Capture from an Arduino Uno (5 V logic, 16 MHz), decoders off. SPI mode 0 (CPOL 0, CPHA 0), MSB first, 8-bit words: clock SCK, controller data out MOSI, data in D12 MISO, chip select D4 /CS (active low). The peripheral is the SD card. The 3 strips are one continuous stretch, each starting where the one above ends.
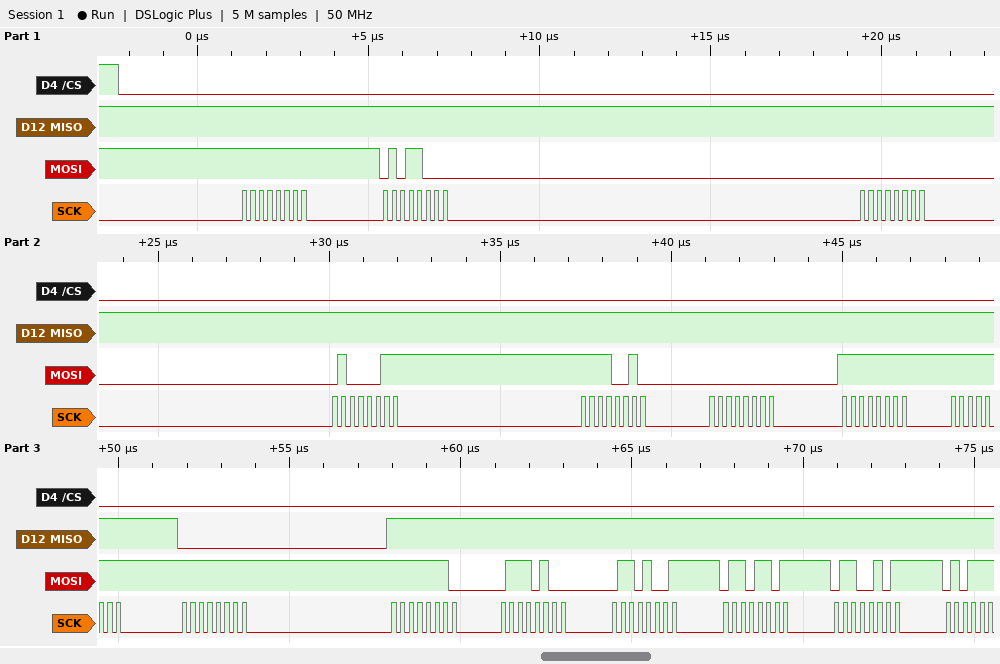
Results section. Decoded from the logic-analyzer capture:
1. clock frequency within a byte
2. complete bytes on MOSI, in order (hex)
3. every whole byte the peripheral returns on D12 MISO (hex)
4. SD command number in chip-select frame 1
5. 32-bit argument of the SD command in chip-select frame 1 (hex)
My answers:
4 MHz
FF 58 00 43 F2 00 FF FF FF FE 74 69 6D 65
FF FF FF FF FF FF FF FF 00 FF FF FF FF FF
CMD24
0x0043F200
